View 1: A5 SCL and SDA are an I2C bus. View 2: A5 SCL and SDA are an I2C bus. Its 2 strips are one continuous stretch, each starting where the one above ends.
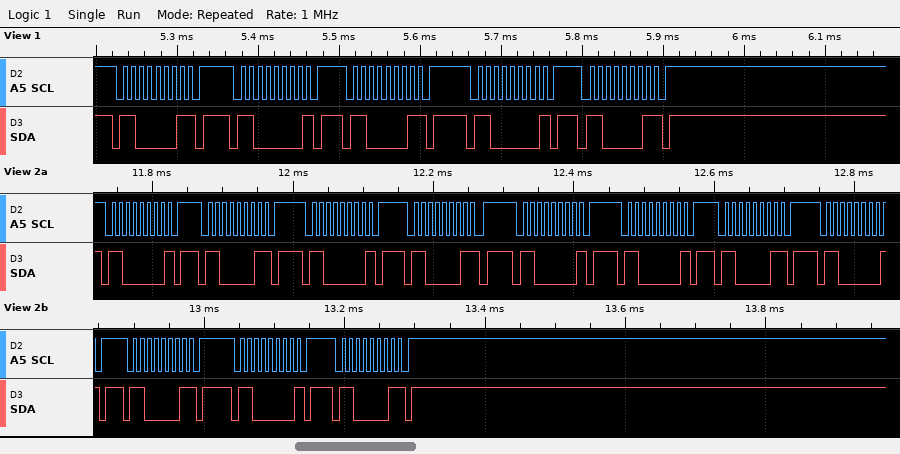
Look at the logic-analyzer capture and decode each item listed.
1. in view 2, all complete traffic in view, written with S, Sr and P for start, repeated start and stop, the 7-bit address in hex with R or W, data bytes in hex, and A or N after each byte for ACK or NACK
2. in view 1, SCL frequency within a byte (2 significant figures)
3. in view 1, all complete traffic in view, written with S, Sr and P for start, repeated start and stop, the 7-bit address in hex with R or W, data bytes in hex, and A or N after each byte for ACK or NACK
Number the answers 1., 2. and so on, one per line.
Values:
1. S 60W N P S 60R N P S 60W N P S 60R N P S 60W N P S 60W N P S 60R N P S 60W N P S 60R N P S 60W N P S 60R N P
2. 100 kHz
3. S 60R N P S 60W N P S 60R N P S 60W N P S 60R N P
